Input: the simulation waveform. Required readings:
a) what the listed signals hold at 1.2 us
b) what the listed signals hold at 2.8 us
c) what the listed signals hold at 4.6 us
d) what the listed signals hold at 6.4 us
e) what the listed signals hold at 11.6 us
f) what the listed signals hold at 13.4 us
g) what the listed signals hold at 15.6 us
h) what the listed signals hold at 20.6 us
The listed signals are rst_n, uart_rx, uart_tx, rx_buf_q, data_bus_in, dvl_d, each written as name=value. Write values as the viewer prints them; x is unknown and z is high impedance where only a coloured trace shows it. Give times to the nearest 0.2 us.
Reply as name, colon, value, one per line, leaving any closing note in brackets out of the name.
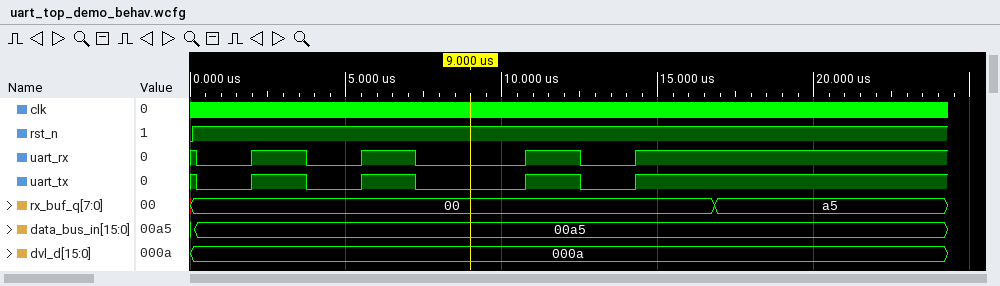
what the listed signals hold at 1.2 us: rst_n=1, uart_rx=0, uart_tx=0, rx_buf_q=00, data_bus_in=00a5, dvl_d=000a
what the listed signals hold at 2.8 us: rst_n=1, uart_rx=1, uart_tx=1, rx_buf_q=00, data_bus_in=00a5, dvl_d=000a
what the listed signals hold at 4.6 us: rst_n=1, uart_rx=0, uart_tx=0, rx_buf_q=00, data_bus_in=00a5, dvl_d=000a
what the listed signals hold at 6.4 us: rst_n=1, uart_rx=1, uart_tx=1, rx_buf_q=00, data_bus_in=00a5, dvl_d=000a
what the listed signals hold at 11.6 us: rst_n=1, uart_rx=1, uart_tx=1, rx_buf_q=00, data_bus_in=00a5, dvl_d=000a
what the listed signals hold at 13.4 us: rst_n=1, uart_rx=0, uart_tx=0, rx_buf_q=00, data_bus_in=00a5, dvl_d=000a
what the listed signals hold at 15.6 us: rst_n=1, uart_rx=1, uart_tx=1, rx_buf_q=00, data_bus_in=00a5, dvl_d=000a
what the listed signals hold at 20.6 us: rst_n=1, uart_rx=1, uart_tx=1, rx_buf_q=a5, data_bus_in=00a5, dvl_d=000a
